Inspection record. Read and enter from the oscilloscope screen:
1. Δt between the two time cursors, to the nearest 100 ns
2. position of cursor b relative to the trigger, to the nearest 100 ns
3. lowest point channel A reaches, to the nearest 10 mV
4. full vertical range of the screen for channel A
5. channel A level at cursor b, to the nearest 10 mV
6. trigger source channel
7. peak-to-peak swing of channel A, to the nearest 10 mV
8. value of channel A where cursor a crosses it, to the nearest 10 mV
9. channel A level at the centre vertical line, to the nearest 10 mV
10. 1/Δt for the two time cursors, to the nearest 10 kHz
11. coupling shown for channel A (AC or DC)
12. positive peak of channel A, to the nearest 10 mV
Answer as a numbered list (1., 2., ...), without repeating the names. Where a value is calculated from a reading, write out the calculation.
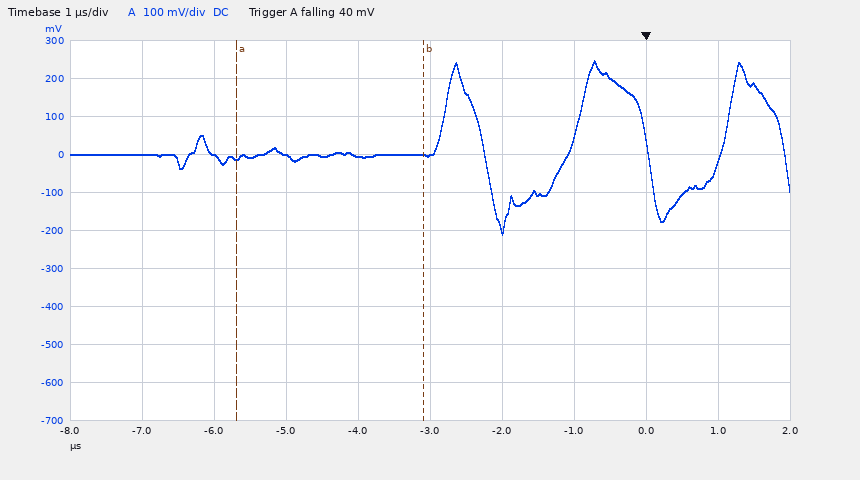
1. 2.6 µs
2. -3.1 µs
3. -210 mV
4. 1 V
5. 0 mV
6. channel A
7. 250 mV − (-210 mV) = 460 mV
8. -10 mV
9. 0 mV
10. 1 / 2.6 µs ≈ 380 kHz
11. DC
12. 250 mV
